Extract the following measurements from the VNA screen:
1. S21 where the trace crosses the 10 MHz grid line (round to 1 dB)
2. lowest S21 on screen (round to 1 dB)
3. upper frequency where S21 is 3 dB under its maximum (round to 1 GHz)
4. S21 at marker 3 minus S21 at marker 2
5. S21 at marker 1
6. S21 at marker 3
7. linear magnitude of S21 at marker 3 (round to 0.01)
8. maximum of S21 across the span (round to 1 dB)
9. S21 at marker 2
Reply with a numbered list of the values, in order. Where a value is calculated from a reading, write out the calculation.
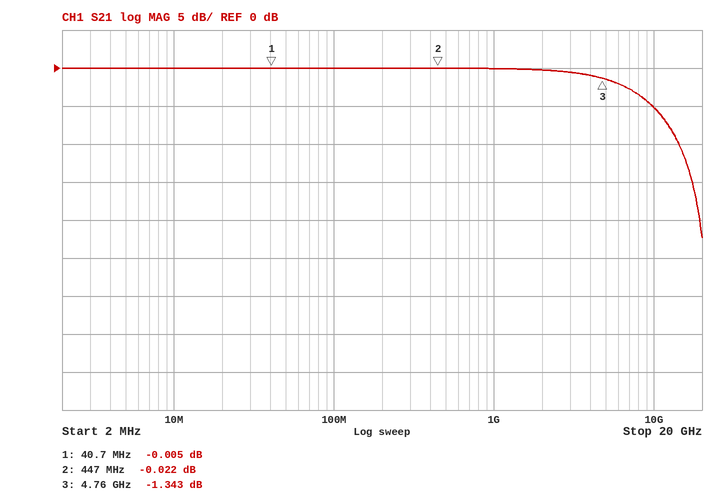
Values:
1. 0 dB
2. -22 dB
3. 7 GHz
4. -1.343 − (-0.022) = -1.321 dB
5. -0.005 dB
6. -1.343 dB
7. 10^(-1.343/20) ≈ 0.86
8. 0 dB
9. -0.022 dB
